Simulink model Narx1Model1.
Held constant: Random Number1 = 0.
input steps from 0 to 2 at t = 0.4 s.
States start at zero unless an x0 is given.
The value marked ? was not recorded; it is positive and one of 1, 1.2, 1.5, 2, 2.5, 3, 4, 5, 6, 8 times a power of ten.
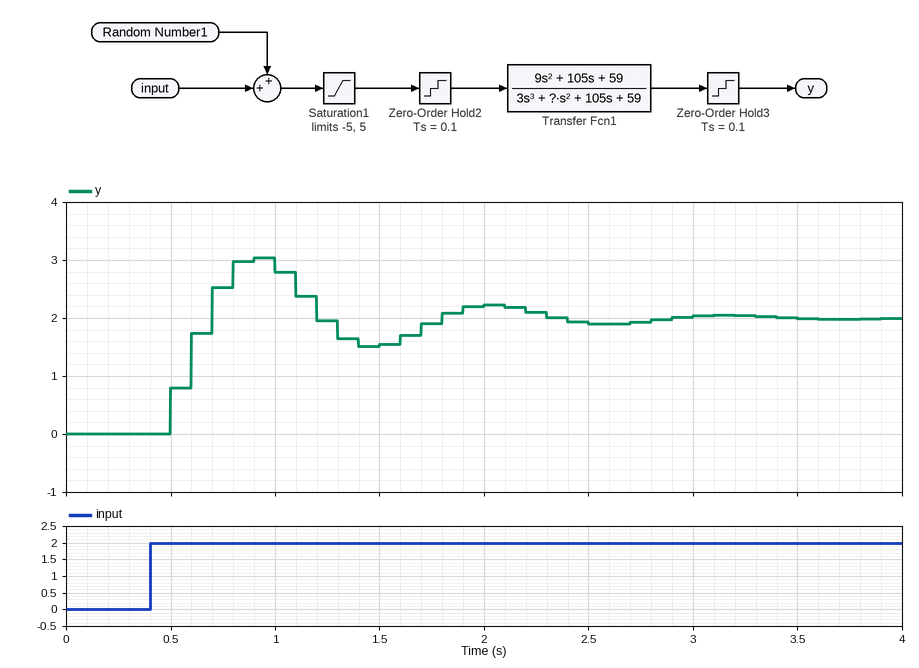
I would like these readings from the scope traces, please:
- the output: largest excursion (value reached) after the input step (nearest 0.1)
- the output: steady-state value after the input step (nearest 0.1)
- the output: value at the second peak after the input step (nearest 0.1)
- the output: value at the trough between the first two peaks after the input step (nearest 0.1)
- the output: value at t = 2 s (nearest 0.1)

3.0
2.0
2.2
1.5
2.2
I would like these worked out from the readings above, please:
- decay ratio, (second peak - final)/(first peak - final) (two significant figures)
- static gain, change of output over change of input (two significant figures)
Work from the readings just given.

0.20
1.0
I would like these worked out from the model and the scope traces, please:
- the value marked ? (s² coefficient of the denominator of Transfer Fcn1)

10
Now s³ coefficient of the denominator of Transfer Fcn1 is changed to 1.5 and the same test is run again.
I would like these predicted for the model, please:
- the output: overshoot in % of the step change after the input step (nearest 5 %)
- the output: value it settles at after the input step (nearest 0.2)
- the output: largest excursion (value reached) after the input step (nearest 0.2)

40 %
2.0
2.8
